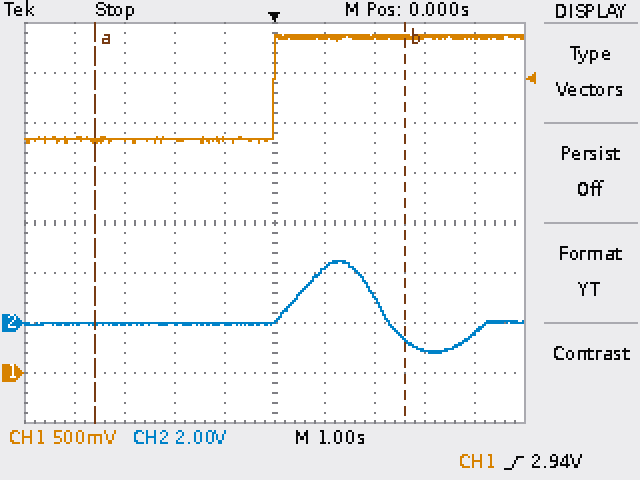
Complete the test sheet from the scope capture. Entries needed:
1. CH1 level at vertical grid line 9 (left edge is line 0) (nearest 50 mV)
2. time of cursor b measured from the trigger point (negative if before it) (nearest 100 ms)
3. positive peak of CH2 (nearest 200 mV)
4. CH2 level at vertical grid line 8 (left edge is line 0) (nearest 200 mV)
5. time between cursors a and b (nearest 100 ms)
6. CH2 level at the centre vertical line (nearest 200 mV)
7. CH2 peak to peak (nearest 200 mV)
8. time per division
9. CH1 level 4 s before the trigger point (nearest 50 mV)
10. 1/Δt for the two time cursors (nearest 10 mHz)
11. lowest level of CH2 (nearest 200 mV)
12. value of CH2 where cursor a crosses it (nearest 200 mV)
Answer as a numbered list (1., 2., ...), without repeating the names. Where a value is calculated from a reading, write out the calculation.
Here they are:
1. 3.35 V
2. +2.6 s
3. 2.4 V
4. -1.0 V
5. 6.2 s
6. 0.0 V
7. 2.4 V − (-1.2 V) = 3.6 V
8. 1 s
9. 2.35 V
10. 1 / 6.2 s ≈ 160 mHz
11. -1.2 V
12. 0.0 V
